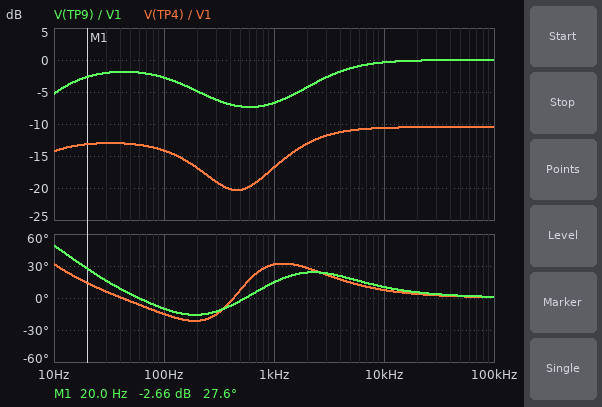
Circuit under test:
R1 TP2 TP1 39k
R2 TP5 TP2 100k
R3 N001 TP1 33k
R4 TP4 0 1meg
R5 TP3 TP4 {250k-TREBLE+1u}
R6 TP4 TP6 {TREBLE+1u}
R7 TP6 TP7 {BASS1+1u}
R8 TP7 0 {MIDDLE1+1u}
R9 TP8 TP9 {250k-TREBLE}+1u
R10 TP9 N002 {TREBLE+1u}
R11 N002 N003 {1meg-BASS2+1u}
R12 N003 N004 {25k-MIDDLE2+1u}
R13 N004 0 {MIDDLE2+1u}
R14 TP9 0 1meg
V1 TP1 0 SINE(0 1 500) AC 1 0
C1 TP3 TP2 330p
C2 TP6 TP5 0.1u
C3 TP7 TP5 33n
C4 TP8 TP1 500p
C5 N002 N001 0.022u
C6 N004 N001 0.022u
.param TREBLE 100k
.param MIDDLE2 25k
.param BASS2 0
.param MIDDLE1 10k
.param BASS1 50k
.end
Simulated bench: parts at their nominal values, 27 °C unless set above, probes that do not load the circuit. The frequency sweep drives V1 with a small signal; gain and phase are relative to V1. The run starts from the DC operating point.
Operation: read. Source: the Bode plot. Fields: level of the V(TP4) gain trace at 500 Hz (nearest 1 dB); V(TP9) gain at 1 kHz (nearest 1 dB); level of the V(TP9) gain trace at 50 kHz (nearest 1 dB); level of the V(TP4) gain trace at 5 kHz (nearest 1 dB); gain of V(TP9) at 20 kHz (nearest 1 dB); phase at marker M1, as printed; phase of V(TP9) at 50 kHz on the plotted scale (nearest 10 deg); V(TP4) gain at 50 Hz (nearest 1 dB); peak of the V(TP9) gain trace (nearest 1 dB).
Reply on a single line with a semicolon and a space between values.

-20 dB; -7 dB; 0 dB; -11 dB; 0 dB; 27.6 deg; 0 deg; -13 dB; 0 dB
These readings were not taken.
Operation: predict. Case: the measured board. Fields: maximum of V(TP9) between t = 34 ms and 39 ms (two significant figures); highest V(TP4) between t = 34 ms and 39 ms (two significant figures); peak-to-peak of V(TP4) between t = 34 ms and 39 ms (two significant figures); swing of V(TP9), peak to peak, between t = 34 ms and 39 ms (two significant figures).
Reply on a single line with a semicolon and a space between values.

430 mV; 96 mV; 190 mV; 870 mV
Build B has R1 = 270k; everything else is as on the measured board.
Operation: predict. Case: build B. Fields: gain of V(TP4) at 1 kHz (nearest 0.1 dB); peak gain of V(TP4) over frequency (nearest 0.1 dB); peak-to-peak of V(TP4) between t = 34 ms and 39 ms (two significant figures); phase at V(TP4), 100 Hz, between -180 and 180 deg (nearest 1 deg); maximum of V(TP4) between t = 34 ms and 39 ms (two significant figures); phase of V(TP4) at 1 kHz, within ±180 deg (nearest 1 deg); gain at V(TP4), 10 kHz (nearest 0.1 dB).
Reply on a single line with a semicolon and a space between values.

-25.2 dB; -19.8 dB; 76 mV; -20 deg; 38 mV; 27 deg; -19.9 dB
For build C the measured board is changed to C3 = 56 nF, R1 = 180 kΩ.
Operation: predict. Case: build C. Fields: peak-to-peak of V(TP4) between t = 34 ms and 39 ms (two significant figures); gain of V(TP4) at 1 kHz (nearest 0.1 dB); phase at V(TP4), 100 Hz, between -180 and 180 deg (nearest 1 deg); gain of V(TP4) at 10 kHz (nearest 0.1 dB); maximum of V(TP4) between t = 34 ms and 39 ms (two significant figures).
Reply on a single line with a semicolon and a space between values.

94 mV; -22.6 dB; -24 deg; -17.4 dB; 47 mV
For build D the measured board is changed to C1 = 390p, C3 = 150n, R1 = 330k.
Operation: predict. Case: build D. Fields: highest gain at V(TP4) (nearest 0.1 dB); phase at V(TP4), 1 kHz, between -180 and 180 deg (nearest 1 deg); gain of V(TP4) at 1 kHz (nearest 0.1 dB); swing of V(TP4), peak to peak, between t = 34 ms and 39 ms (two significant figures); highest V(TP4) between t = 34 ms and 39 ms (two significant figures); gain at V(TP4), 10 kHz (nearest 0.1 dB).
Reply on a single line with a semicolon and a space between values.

-21.2 dB; 33 deg; -25.2 dB; 71 mV; 35 mV; -21.3 dB
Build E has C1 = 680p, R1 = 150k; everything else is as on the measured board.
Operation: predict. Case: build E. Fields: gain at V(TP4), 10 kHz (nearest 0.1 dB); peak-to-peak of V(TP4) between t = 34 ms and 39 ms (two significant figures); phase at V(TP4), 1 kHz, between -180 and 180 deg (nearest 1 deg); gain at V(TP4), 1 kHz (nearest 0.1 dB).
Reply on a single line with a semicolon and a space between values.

-16.2 dB; 170 mV; 20 deg; -18.4 dB
